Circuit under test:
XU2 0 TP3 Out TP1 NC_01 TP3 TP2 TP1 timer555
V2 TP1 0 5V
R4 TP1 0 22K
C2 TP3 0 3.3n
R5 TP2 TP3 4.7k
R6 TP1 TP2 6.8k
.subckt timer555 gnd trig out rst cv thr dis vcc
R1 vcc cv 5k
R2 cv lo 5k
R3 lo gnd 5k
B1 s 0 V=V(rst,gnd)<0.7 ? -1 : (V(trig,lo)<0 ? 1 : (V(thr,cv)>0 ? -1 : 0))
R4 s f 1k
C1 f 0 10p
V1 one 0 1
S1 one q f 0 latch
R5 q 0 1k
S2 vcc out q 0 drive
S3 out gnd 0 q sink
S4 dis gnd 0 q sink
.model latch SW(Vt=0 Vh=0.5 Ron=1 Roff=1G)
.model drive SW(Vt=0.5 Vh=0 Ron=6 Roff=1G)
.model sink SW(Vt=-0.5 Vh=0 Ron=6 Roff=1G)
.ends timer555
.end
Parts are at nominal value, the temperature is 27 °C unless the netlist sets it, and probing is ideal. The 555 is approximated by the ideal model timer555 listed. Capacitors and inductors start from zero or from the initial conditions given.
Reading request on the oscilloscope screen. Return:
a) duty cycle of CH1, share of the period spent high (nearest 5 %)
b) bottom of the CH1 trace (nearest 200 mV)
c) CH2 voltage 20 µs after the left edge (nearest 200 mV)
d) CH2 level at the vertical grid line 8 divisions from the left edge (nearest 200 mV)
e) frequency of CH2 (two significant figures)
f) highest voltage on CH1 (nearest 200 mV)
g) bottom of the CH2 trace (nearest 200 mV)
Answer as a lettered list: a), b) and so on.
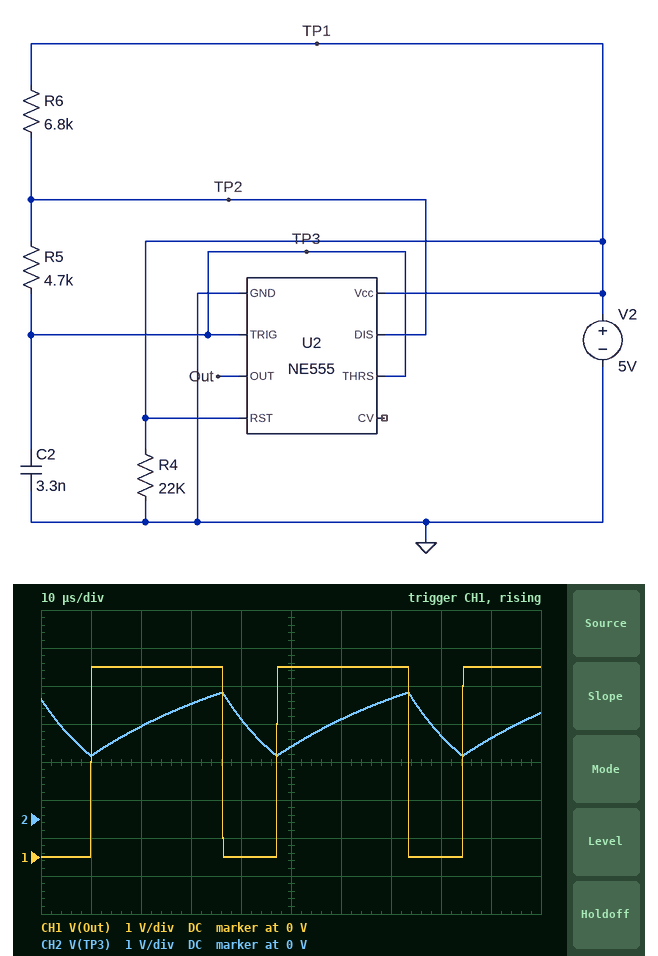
a) 70 %
b) 0 V
c) 2.4 V
d) 2.2 V
e) 27 kHz
f) 5.0 V
g) 1.6 V
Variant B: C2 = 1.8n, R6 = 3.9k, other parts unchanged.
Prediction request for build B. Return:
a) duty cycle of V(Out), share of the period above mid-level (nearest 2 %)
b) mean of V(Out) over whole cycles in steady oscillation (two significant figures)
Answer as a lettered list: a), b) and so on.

a) 64 %
b) 3.2 V
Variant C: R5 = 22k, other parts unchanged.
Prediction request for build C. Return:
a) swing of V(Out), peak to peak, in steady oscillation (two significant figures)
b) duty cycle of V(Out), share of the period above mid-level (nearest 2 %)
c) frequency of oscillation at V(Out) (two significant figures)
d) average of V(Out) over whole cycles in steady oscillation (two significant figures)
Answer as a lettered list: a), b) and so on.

a) 5.0 V
b) 56 %
c) 8.6 kHz
d) 2.8 V
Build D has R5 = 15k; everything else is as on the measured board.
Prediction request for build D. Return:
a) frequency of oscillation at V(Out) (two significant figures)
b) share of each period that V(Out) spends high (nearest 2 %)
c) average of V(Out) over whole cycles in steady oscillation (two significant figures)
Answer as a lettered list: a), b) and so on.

a) 12 kHz
b) 60 %
c) 3.0 V
